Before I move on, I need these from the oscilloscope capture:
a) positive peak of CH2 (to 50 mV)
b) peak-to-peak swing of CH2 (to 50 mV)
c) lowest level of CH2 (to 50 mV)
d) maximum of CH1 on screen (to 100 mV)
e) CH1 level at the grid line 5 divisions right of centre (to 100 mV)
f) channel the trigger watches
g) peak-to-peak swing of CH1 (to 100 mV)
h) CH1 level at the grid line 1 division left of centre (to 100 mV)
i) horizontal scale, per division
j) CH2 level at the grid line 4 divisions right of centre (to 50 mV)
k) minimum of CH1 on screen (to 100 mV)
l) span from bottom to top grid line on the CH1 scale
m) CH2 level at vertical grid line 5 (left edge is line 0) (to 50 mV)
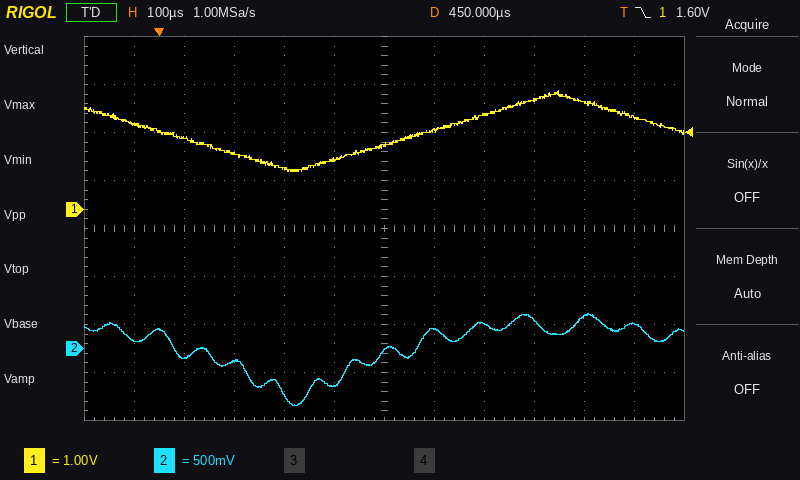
350 mV
950 mV
-600 mV
2.5 V
1.9 V
CH1
1.7 V
1.0 V
100 µs
350 mV
800 mV
8 V
-400 mV
